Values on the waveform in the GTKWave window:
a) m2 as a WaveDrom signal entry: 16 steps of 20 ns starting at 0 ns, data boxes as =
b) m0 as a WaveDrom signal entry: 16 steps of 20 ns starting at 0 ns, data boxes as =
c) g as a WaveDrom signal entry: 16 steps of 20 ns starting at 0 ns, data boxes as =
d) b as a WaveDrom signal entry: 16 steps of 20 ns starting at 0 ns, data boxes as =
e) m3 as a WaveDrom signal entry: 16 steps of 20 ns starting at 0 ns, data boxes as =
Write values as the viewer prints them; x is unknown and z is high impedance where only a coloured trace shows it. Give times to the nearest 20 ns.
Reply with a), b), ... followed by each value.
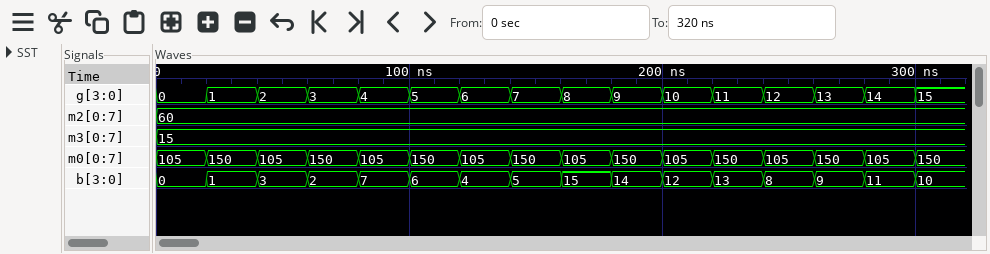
a) {name: 'm2', wave: '=...............', data: '60'}
b) {name: 'm0', wave: '================', data: '105 150 105 150 105 150 105 150 105 150 105 150 105 150 105 150'}
c) {name: 'g', wave: '================', data: '0 1 2 3 4 5 6 7 8 9 10 11 12 13 14 15'}
d) {name: 'b', wave: '================', data: '0 1 3 2 7 6 4 5 15 14 12 13 8 9 11 10'}
e) {name: 'm3', wave: '=...............', data: '15'}
